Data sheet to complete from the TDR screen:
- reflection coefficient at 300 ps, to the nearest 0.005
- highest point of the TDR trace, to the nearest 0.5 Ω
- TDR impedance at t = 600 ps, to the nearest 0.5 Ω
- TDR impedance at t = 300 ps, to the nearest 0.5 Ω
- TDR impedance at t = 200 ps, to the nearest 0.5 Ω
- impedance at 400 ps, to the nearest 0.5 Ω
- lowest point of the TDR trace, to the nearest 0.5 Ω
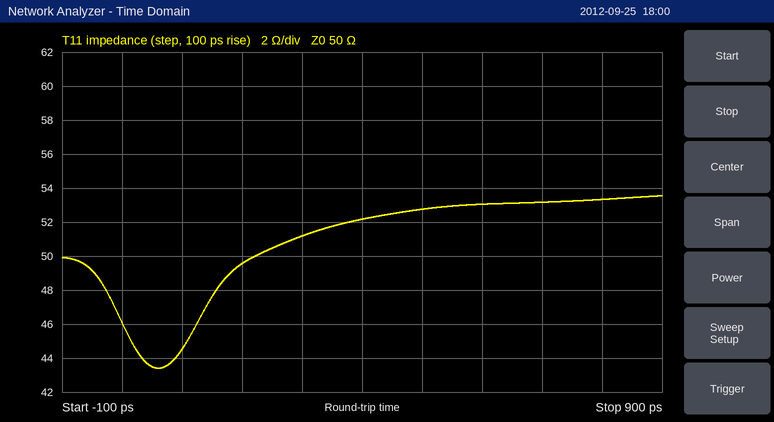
+0.010
53.5 Ω
53.0 Ω
51.0 Ω
49.5 Ω
52.0 Ω
43.5 Ω
